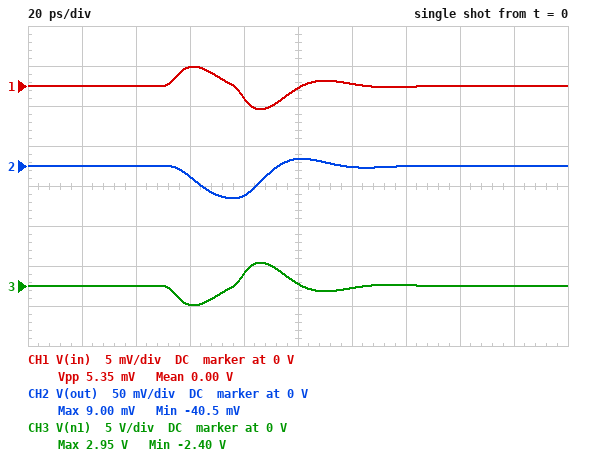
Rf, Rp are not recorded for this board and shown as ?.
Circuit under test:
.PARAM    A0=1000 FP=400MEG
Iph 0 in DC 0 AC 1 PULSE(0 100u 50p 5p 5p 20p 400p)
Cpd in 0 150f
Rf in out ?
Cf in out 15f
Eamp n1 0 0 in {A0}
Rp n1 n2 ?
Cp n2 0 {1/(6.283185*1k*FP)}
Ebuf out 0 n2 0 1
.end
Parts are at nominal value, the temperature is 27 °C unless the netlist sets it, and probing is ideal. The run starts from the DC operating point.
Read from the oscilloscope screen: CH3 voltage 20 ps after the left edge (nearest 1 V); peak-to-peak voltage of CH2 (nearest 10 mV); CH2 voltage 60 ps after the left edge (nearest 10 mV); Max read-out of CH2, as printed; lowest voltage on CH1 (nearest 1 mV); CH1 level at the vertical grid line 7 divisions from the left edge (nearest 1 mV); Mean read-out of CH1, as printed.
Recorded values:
0 V
50 mV
-10 mV
9.00 mV
-3 mV
0 V
0.00 V
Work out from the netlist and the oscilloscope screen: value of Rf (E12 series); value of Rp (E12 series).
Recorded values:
330 Ω
2.2 kΩ
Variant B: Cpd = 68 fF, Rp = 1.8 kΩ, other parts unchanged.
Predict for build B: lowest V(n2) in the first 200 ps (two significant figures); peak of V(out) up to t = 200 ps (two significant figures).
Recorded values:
-35 mV
2.3 mV
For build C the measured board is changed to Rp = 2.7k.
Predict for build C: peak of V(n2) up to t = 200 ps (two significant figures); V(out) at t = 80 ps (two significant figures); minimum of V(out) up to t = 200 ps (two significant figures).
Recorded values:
10 mV
-39 mV
-41 mV
